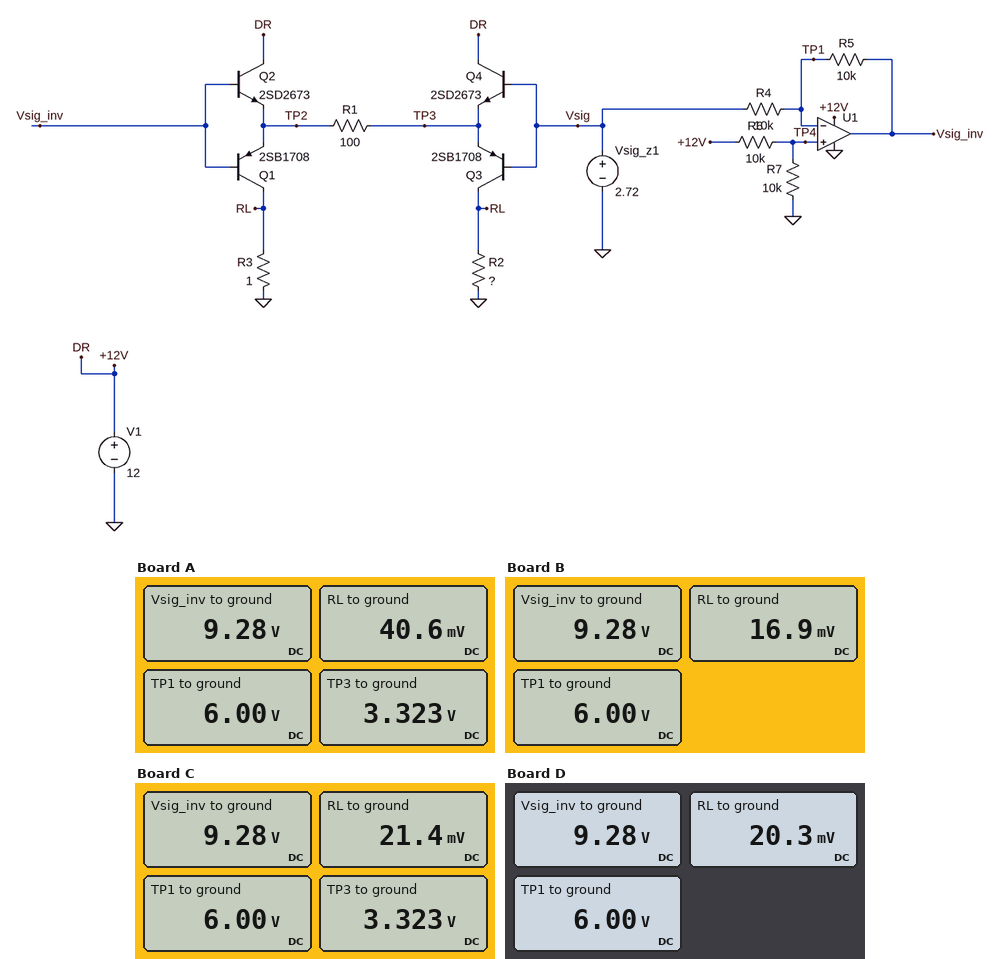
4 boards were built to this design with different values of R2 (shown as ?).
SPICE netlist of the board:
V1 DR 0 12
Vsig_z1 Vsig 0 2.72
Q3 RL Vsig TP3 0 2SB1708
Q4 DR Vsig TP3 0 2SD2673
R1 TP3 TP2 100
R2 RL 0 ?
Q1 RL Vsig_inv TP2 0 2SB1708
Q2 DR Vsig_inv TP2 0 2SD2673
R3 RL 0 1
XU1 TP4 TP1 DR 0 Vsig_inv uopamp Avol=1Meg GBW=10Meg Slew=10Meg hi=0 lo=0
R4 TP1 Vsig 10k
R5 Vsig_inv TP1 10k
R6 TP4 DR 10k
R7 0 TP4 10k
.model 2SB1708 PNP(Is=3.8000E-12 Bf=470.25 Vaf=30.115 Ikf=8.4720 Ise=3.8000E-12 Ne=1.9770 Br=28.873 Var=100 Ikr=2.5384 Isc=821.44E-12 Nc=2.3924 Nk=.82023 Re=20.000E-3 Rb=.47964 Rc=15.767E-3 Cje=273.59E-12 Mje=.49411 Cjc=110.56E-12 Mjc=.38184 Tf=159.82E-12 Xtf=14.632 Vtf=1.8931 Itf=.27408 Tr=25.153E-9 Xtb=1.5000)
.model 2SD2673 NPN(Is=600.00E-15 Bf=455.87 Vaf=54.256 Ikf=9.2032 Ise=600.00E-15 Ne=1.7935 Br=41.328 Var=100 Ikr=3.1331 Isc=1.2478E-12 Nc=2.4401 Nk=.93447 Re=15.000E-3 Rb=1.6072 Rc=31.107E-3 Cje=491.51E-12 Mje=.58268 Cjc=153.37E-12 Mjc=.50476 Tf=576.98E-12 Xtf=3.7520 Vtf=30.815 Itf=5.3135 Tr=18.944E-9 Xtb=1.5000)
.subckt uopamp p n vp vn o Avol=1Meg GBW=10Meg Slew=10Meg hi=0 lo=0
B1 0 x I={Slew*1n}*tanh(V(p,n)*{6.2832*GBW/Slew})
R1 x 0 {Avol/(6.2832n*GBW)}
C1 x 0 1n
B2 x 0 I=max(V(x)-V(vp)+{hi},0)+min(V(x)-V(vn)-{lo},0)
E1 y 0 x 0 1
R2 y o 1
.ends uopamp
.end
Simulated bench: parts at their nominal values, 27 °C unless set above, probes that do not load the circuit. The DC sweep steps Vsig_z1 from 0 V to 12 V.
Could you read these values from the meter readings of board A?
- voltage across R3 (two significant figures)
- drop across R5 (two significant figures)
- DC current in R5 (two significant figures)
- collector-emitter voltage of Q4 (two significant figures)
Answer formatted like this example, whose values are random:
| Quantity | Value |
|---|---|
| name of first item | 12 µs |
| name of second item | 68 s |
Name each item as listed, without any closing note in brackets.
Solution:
| Quantity | Value |
|---|---|
| voltage across R3 | 41 mV |
| drop across R5 | 3.3 V |
| DC current in R5 | 330 µA |
| collector-emitter voltage of Q4 | 8.7 V |
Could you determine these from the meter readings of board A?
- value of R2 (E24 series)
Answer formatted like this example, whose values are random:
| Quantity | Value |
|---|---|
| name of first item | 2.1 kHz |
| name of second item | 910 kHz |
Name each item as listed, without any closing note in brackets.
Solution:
| Quantity | Value |
|---|---|
| value of R2 | 3.3 Ω |
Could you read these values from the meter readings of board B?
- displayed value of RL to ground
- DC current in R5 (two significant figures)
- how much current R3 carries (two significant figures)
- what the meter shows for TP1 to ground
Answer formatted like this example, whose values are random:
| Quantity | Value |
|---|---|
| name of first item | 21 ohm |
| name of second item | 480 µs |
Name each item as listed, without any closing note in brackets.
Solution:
| Quantity | Value |
|---|---|
| displayed value of RL to ground | 16.9 mV |
| DC current in R5 | 330 µA |
| how much current R3 carries | 17 mA |
| what the meter shows for TP1 to ground | 6.00 V |
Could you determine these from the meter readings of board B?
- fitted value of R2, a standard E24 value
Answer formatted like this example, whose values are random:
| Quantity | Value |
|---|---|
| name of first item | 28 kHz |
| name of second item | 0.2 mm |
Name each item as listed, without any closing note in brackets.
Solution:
| Quantity | Value |
|---|---|
| fitted value of R2, a standard E24 value | 0.47 Ω |
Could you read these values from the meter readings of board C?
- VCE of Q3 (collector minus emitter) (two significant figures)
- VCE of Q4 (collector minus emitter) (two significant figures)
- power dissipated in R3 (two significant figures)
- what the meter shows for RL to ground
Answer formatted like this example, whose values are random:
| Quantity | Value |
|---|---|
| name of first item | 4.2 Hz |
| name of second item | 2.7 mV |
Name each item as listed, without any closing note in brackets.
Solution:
| Quantity | Value |
|---|---|
| VCE of Q3 (collector minus emitter) | -3.3 V |
| VCE of Q4 (collector minus emitter) | 8.7 V |
| power dissipated in R3 | 460 µW |
| what the meter shows for RL to ground | 21.4 mV |
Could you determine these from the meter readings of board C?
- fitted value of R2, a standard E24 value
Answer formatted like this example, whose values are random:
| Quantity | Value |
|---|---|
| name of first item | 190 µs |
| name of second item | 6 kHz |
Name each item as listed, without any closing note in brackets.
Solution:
| Quantity | Value |
|---|---|
| fitted value of R2, a standard E24 value | 0.68 Ω |
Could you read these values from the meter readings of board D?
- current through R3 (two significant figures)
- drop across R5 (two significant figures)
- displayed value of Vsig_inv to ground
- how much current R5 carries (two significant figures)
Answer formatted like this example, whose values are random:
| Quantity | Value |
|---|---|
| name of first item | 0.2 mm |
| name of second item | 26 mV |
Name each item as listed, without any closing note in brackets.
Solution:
| Quantity | Value |
|---|---|
| current through R3 | 20 mA |
| drop across R5 | 3.3 V |
| displayed value of Vsig_inv to ground | 9.28 V |
| how much current R5 carries | 330 µA |
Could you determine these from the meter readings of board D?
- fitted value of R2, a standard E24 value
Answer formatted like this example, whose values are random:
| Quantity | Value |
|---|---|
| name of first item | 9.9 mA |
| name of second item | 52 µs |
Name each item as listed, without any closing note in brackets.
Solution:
| Quantity | Value |
|---|---|
| fitted value of R2, a standard E24 value | 0.62 Ω |
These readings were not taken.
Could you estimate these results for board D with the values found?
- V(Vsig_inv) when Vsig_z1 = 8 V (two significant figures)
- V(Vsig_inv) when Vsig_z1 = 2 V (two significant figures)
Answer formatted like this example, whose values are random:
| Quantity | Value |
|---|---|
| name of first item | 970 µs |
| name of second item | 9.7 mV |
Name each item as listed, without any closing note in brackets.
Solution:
| Quantity | Value |
|---|---|
| V(Vsig_inv) when Vsig_z1 = 8 V | 4.0 V |
| V(Vsig_inv) when Vsig_z1 = 2 V | 10 V |
